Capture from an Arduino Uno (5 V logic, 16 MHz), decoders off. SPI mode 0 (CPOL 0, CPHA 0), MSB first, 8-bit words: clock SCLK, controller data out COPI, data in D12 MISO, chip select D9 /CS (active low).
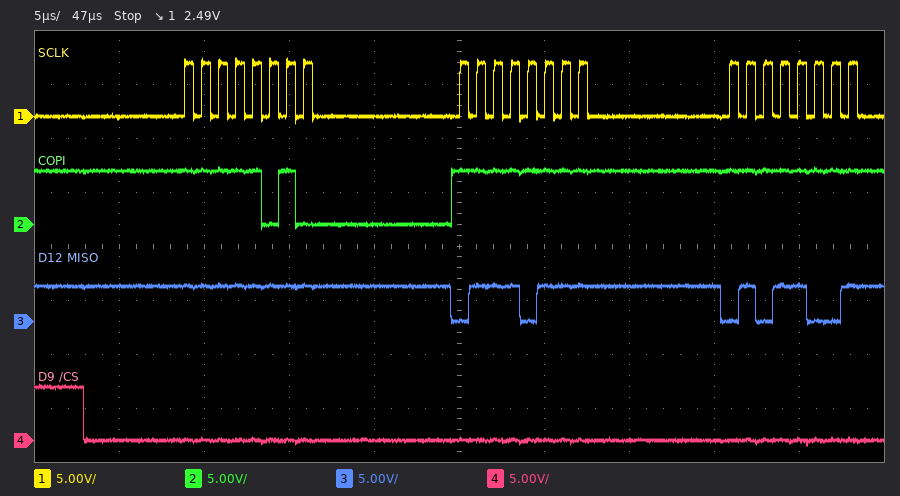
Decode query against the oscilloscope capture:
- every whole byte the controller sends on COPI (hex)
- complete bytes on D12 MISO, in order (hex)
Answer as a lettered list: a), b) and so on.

a) 0xFA 0xFF 0xFF
b) 0xFF 0x77 0x59
